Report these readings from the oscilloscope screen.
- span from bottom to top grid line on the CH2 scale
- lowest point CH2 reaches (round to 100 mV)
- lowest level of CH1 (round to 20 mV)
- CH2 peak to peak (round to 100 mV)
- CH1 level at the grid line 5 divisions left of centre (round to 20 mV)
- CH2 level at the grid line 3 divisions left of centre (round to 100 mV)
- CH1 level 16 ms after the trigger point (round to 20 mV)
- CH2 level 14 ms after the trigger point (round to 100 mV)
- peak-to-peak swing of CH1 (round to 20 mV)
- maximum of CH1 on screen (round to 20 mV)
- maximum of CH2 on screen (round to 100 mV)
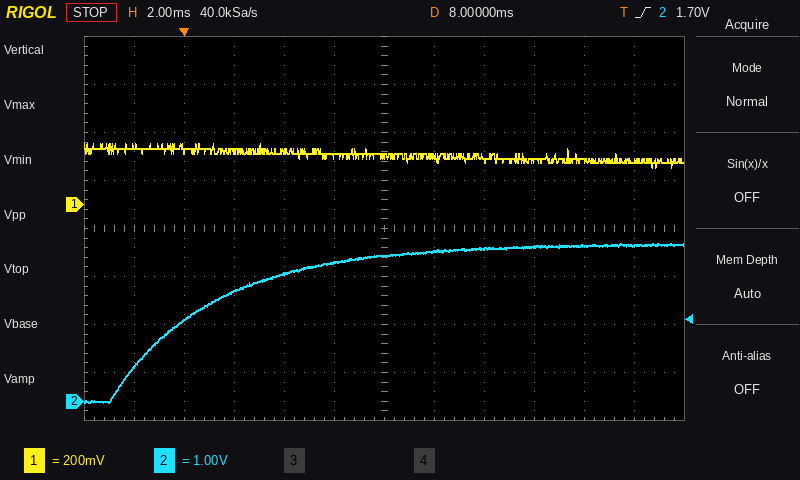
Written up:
8 V
0.0 V
160 mV
3.3 V
240 mV
2.3 V
180 mV
3.2 V
100 mV
260 mV
3.3 V
